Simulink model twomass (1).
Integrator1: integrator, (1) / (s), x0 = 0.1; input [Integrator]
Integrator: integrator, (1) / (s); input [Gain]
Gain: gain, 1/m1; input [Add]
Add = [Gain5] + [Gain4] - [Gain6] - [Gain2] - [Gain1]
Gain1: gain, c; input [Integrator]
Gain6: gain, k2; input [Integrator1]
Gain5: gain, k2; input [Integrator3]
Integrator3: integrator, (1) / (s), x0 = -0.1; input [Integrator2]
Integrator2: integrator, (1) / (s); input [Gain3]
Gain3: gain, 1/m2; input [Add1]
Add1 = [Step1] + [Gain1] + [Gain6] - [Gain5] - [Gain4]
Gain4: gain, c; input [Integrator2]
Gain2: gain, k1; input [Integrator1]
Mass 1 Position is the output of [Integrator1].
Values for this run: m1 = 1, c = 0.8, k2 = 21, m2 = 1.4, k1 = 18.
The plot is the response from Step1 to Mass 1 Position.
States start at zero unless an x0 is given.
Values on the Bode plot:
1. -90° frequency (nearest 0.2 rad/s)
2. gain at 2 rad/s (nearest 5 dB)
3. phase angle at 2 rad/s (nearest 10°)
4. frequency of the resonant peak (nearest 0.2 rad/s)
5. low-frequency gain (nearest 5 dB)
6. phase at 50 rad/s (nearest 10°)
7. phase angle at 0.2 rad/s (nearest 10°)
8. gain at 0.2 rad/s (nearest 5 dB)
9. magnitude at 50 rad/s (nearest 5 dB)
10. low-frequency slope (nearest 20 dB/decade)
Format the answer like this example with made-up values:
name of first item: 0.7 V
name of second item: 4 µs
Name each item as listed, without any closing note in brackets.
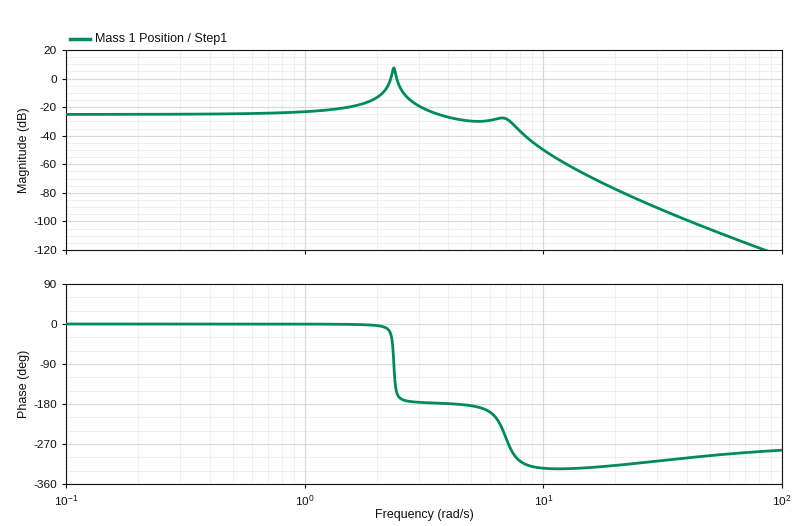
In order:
-90° frequency: 2.4 rad/s
gain at 2 rad/s: -15 dB
phase angle at 2 rad/s: 0°
frequency of the resonant peak: 2.4 rad/s
low-frequency gain: -25 dB
phase at 50 rad/s: -300°
phase angle at 0.2 rad/s: 0°
gain at 0.2 rad/s: -25 dB
magnitude at 50 rad/s: -105 dB
low-frequency slope: 0 dB/decade
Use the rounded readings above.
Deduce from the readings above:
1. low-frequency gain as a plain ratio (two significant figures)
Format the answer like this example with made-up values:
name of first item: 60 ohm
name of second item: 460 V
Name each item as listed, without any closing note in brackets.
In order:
low-frequency gain as a plain ratio: 0.056
